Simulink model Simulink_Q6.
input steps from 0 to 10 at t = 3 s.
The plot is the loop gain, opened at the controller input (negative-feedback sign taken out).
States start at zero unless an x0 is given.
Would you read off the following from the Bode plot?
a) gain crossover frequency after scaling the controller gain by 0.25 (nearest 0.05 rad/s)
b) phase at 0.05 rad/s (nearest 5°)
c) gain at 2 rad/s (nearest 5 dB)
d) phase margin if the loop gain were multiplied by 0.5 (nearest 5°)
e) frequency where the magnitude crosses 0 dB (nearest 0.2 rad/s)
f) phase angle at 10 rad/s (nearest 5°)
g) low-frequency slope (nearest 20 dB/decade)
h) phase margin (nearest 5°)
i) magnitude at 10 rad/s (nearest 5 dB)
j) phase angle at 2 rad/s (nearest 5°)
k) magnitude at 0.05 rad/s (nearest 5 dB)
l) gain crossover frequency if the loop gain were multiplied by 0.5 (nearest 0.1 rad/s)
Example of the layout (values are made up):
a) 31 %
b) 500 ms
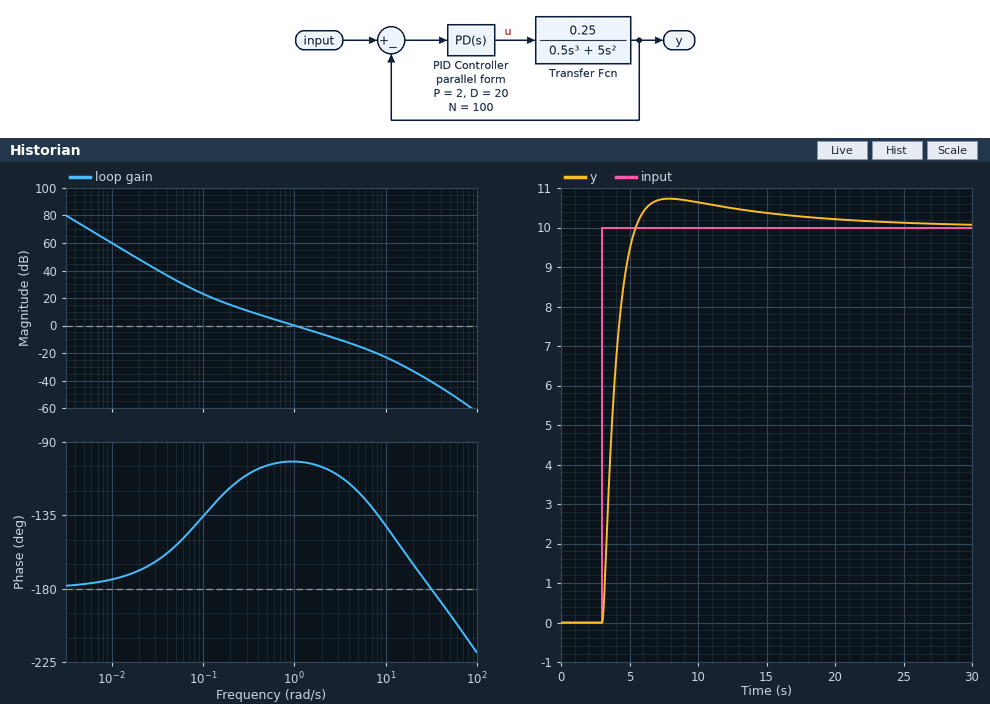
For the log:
a) 0.25 rad/s
b) -155°
c) -5 dB
d) 75°
e) 1.0 rad/s
f) -140°
g) -40 dB/decade
h) 80°
i) -25 dB
j) -105°
k) 35 dB
l) 0.5 rad/s
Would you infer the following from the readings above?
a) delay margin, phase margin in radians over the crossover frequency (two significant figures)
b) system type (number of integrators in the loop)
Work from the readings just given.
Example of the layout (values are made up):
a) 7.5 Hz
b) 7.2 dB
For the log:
a) 1.4 s
b) 2
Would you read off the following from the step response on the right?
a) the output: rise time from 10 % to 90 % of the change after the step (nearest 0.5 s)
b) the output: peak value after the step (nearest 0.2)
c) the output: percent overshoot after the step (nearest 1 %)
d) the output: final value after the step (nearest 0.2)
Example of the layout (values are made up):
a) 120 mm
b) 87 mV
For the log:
a) 1.5 s
b) 10.8
c) 7 %
d) 10.0
